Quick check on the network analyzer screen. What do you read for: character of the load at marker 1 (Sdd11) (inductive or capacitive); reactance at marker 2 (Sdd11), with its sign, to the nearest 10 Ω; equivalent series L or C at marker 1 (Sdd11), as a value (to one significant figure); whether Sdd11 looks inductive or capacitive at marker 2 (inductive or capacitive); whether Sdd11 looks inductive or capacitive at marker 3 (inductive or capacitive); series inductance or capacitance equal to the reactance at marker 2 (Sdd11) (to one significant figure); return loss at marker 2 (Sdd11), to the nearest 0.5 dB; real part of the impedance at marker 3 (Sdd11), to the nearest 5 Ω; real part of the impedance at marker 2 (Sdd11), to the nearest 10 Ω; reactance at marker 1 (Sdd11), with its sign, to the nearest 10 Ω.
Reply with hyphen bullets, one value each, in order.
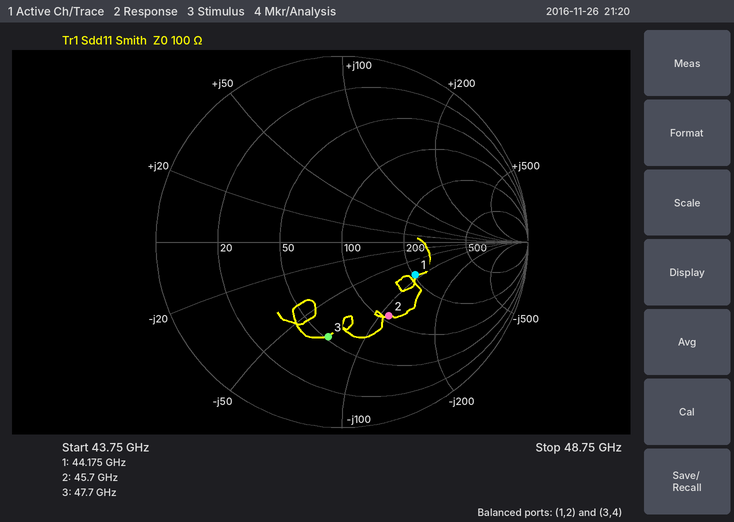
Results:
- capacitive
- -110 Ω
- 40 fF
- capacitive
- capacitive
- 30 fF
- 6.5 dB
- 50 Ω
- 110 Ω
- -90 Ω
